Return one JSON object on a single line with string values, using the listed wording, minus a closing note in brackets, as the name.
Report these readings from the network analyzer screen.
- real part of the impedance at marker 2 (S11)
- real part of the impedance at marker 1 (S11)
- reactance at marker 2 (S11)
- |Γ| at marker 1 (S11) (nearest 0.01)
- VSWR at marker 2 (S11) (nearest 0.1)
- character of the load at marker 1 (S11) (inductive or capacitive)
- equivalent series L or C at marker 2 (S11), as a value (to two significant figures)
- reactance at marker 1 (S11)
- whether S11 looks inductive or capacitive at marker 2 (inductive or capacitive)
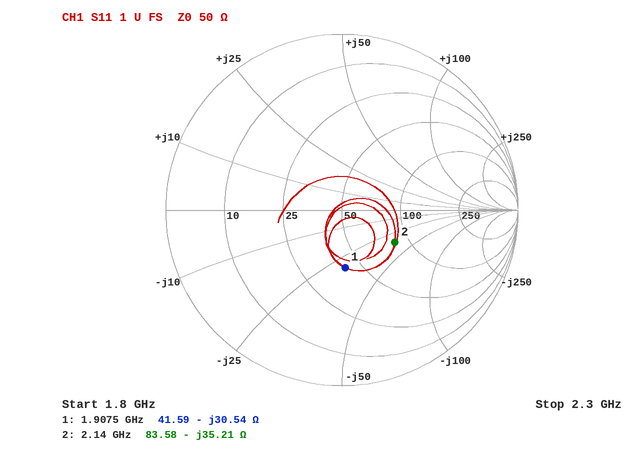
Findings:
{"real part of the impedance at marker 2": "83.58 Ω", "real part of the impedance at marker 1": "41.59 Ω", "reactance at marker 2": "-35.21 Ω", "|Γ| at marker 1 (S11)": "0.33", "VSWR at marker 2 (S11)": "2.1", "character of the load at marker 1 (S11)": "capacitive", "equivalent series L or C at marker 2 (S11), as a value": "2.1 pF", "reactance at marker 1": "-30.54 Ω", "whether S11 looks inductive or capacitive at marker 2": "capacitive"}
